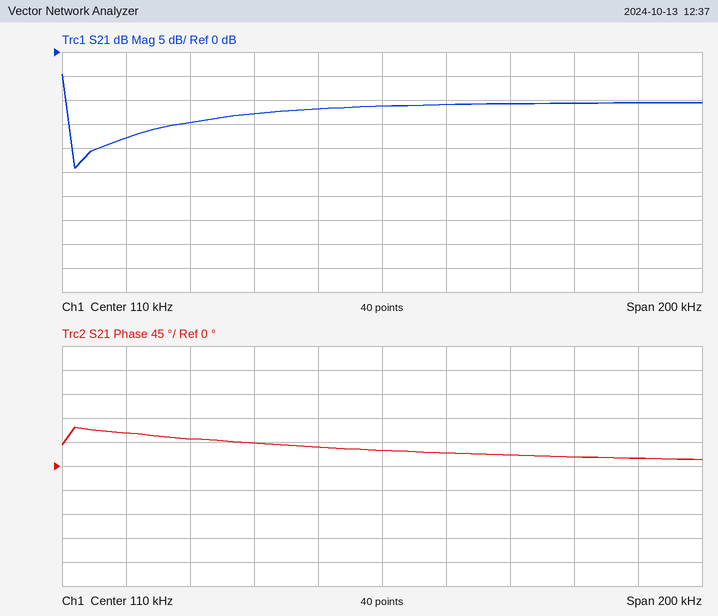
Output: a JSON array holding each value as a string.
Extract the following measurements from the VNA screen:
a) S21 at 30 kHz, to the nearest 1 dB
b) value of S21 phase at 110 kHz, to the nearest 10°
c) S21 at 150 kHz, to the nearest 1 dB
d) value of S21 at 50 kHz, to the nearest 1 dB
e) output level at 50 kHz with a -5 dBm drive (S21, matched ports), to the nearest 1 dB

["-18 dB", "30°", "-11 dB", "-15 dB", "-20 dBm"]
